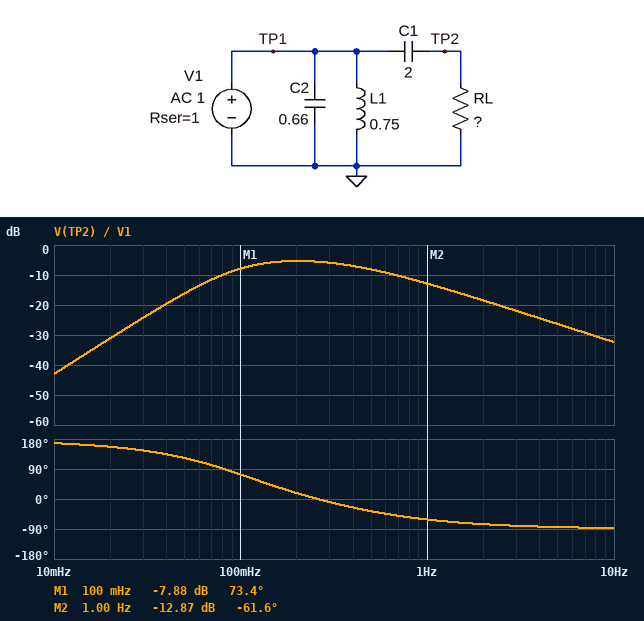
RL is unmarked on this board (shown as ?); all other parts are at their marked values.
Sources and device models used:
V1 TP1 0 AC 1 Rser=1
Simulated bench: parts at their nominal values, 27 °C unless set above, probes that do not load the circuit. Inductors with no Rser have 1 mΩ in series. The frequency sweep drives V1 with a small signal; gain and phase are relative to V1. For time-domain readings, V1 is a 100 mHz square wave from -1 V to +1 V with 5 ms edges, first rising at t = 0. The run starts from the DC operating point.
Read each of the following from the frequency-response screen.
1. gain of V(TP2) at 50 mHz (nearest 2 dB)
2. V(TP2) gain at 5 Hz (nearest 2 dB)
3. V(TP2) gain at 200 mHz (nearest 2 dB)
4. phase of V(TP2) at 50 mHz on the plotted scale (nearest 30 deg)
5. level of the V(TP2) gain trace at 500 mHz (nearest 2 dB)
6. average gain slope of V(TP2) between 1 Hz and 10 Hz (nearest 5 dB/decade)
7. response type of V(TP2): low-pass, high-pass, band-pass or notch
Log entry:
-16 dB
-26 dB
-6 dB
120 deg
-8 dB
-20 dB/decade
band-pass
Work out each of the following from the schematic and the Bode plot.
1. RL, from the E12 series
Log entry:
1.2 Ω
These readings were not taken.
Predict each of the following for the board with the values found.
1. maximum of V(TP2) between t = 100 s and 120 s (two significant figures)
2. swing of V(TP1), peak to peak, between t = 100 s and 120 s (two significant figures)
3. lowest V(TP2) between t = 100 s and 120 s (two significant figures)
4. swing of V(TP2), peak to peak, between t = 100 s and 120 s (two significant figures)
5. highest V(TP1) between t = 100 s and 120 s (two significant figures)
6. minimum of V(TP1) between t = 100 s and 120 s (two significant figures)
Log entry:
840 mV
1.7 V
-840 mV
1.7 V
870 mV
-870 mV
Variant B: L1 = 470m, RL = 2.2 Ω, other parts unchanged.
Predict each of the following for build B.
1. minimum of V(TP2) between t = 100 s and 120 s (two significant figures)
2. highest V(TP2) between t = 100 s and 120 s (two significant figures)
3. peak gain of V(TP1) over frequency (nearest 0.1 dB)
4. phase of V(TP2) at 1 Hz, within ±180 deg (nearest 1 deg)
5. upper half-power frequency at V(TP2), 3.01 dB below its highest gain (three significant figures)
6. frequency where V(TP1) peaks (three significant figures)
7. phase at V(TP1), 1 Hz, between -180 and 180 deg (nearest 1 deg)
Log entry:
-820 mV
820 mV
-3.2 dB
-67 deg
506 mHz
278 mHz
-69 deg
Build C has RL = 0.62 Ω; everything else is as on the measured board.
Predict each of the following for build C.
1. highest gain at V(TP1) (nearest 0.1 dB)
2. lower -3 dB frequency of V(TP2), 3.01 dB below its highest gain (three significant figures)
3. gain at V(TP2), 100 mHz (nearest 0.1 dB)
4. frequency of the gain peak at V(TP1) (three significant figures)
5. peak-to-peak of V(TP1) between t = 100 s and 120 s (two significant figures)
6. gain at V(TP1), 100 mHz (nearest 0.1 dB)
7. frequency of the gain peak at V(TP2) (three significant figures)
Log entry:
-5.2 dB
86.9 mHz
-9.6 dB
115 mHz
1.6 V
-5.4 dB
152 mHz
